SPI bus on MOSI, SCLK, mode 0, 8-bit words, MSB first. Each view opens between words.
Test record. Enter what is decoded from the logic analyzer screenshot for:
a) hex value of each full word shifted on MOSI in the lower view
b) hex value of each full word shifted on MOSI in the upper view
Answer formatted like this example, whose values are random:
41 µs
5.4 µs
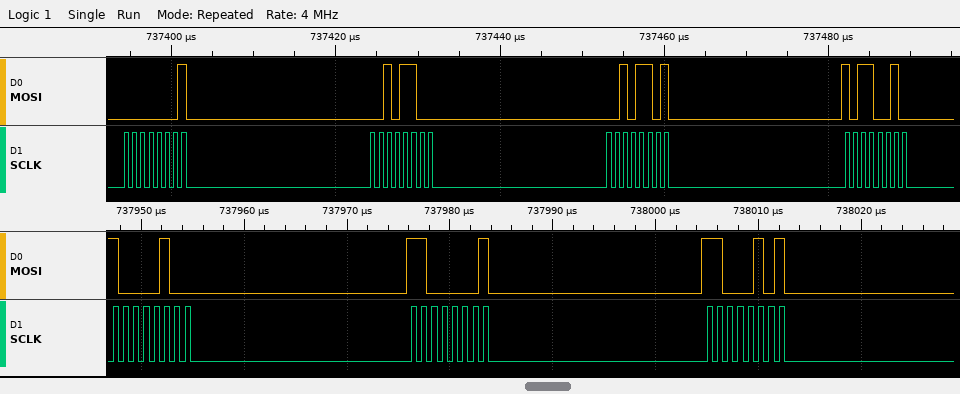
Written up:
84, C1, C5
01, 2C, 2D, B2
